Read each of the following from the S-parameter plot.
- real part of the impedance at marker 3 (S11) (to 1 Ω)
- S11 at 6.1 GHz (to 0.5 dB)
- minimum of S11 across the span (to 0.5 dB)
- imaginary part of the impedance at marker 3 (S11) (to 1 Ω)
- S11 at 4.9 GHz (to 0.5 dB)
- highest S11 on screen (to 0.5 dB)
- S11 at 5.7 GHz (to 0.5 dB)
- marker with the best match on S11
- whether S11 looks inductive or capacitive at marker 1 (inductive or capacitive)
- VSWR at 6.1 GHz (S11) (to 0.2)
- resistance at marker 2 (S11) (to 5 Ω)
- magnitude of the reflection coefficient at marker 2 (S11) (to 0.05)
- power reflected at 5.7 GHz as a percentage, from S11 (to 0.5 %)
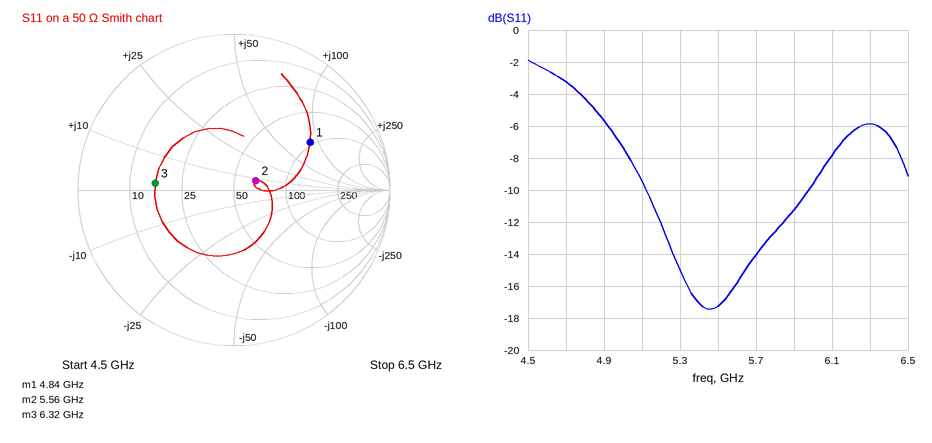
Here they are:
16 Ω
-8.0 dB
-17.5 dB
+2 Ω
-5.5 dB
-2.0 dB
-14.0 dB
marker 2
inductive
2.4
65 Ω
0.15
4.0 %
